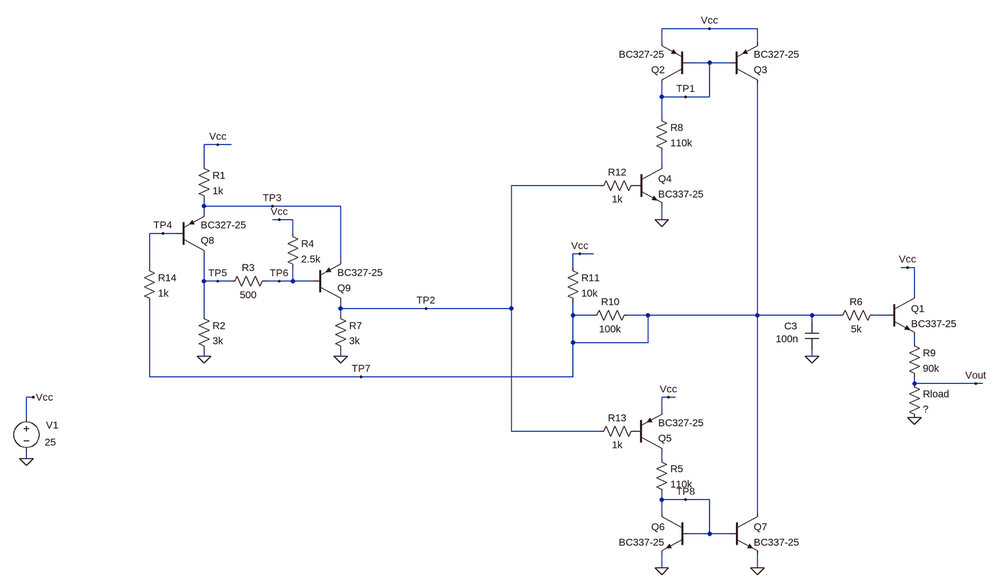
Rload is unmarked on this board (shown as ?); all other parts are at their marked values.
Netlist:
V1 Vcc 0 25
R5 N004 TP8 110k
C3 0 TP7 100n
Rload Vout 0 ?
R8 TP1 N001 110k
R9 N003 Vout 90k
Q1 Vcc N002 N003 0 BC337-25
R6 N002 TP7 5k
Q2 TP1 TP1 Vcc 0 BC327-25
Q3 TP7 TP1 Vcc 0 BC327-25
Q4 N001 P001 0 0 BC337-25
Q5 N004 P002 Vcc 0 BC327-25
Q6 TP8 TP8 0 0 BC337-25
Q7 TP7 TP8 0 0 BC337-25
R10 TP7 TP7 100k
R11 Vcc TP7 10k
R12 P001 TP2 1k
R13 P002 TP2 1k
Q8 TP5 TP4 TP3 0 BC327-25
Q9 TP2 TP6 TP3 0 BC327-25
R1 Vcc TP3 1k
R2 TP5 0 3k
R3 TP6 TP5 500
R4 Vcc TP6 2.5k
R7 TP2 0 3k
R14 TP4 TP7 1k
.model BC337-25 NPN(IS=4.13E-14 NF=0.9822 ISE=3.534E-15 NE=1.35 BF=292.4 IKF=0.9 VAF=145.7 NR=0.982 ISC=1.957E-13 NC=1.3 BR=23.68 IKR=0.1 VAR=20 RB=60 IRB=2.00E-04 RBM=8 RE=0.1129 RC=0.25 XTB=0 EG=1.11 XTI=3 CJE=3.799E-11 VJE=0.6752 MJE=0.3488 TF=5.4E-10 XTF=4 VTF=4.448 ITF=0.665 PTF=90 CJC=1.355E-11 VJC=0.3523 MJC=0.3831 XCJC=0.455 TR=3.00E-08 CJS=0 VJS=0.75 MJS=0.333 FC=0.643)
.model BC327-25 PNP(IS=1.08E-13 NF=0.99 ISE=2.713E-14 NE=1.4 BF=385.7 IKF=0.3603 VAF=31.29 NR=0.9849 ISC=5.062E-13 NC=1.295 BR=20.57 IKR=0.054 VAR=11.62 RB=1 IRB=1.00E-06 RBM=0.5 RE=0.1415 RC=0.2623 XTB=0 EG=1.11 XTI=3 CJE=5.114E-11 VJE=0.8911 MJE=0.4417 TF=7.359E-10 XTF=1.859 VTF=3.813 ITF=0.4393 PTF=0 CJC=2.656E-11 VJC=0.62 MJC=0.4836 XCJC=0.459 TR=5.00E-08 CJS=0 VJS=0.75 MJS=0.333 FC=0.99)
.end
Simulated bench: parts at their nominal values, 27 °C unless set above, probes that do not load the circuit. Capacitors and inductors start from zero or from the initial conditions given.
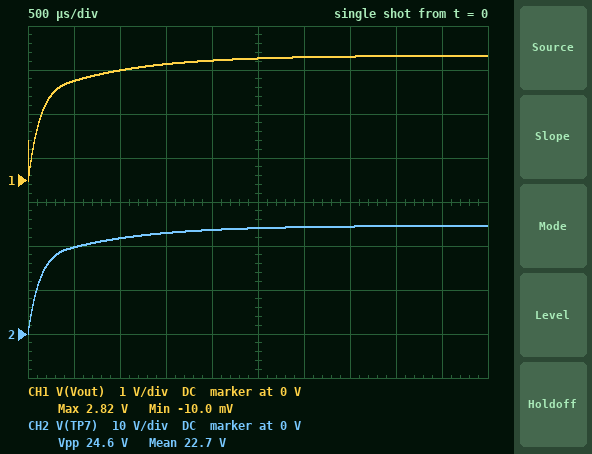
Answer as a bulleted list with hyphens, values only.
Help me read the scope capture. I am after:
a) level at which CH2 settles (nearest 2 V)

- 24 V
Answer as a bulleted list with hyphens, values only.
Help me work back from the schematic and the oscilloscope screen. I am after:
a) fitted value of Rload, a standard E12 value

- 12 kΩ
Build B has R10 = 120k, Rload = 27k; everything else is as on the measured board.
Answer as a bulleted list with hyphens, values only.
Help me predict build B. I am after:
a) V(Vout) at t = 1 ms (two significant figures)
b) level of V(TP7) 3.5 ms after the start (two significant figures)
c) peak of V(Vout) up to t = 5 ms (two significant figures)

- 4.9 V
- 24 V
- 5.5 V
